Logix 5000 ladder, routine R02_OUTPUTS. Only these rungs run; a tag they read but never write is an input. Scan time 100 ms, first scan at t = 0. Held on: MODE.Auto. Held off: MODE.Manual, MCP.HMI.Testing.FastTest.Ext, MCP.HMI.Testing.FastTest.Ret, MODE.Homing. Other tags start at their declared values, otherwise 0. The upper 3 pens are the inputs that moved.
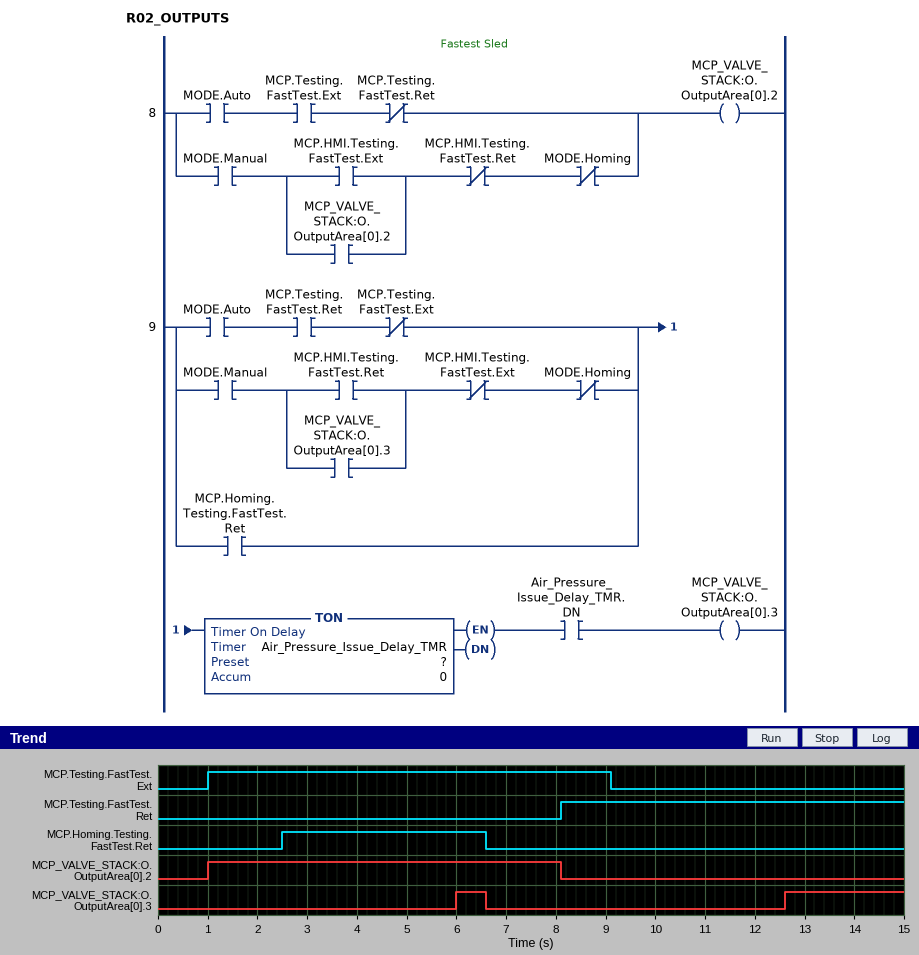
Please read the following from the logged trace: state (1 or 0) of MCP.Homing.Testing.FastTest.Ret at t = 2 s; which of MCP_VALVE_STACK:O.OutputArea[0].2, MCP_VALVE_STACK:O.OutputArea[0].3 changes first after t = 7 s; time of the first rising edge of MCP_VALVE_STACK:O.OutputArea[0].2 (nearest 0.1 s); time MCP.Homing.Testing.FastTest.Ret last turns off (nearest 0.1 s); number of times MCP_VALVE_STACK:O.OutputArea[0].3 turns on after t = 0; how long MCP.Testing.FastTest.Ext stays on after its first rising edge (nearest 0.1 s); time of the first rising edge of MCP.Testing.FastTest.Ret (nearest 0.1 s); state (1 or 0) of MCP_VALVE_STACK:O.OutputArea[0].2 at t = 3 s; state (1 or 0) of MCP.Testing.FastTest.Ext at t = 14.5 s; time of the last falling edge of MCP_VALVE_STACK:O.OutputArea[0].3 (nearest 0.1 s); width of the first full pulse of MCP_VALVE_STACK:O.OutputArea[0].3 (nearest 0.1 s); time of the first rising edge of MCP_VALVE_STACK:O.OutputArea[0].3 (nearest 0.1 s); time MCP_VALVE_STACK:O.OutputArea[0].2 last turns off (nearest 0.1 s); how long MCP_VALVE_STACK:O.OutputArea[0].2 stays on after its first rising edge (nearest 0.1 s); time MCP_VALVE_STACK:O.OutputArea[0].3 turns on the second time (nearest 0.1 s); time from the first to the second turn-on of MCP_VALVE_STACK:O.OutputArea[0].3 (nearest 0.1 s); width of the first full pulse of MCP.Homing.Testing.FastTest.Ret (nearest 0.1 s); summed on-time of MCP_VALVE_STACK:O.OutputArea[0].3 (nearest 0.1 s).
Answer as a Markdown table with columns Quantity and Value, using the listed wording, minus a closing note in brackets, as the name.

| Quantity | Value |
|---|---|
| state (1 or 0) of MCP.Homing.Testing.FastTest.Ret at t = 2 s | 0 |
| which of MCP_VALVE_STACK:O.OutputArea[0].2, MCP_VALVE_STACK:O.OutputArea[0].3 changes first after t = 7 s | MCP_VALVE_STACK:O.OutputArea[0].2 |
| time of the first rising edge of MCP_VALVE_STACK:O.OutputArea[0].2 | 1.0 s |
| time MCP.Homing.Testing.FastTest.Ret last turns off | 6.6 s |
| number of times MCP_VALVE_STACK:O.OutputArea[0].3 turns on after t = 0 | 2 |
| how long MCP.Testing.FastTest.Ext stays on after its first rising edge | 8.1 s |
| time of the first rising edge of MCP.Testing.FastTest.Ret | 8.1 s |
| state (1 or 0) of MCP_VALVE_STACK:O.OutputArea[0].2 at t = 3 s | 1 |
| state (1 or 0) of MCP.Testing.FastTest.Ext at t = 14.5 s | 0 |
| time of the last falling edge of MCP_VALVE_STACK:O.OutputArea[0].3 | 6.6 s |
| width of the first full pulse of MCP_VALVE_STACK:O.OutputArea[0].3 | 0.6 s |
| time of the first rising edge of MCP_VALVE_STACK:O.OutputArea[0].3 | 6.0 s |
| time MCP_VALVE_STACK:O.OutputArea[0].2 last turns off | 8.1 s |
| how long MCP_VALVE_STACK:O.OutputArea[0].2 stays on after its first rising edge | 7.1 s |
| time MCP_VALVE_STACK:O.OutputArea[0].3 turns on the second time | 12.6 s |
| time from the first to the second turn-on of MCP_VALVE_STACK:O.OutputArea[0].3 | 6.6 s |
| width of the first full pulse of MCP.Homing.Testing.FastTest.Ret | 4.1 s |
| summed on-time of MCP_VALVE_STACK:O.OutputArea[0].3 | 3.0 s |
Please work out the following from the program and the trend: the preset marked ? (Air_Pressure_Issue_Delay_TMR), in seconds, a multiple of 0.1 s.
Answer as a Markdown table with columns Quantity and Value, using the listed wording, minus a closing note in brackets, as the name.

| Quantity | Value |
|---|---|
| the preset marked ? (Air_Pressure_Issue_Delay_TMR), in seconds, a multiple of 0.1 s | 3.5 s |
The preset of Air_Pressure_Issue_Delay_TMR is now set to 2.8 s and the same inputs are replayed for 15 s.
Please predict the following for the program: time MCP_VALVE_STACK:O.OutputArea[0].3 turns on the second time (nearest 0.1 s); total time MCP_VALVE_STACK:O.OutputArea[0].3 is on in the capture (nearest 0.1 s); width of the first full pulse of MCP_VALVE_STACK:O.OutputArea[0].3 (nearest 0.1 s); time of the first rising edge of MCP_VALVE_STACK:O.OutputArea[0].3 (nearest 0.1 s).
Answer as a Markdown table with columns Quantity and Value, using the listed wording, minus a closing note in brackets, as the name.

| Quantity | Value |
|---|---|
| time MCP_VALVE_STACK:O.OutputArea[0].3 turns on the second time | 11.9 s |
| total time MCP_VALVE_STACK:O.OutputArea[0].3 is on in the capture | 4.4 s |
| width of the first full pulse of MCP_VALVE_STACK:O.OutputArea[0].3 | 1.3 s |
| time of the first rising edge of MCP_VALVE_STACK:O.OutputArea[0].3 | 5.3 s |
